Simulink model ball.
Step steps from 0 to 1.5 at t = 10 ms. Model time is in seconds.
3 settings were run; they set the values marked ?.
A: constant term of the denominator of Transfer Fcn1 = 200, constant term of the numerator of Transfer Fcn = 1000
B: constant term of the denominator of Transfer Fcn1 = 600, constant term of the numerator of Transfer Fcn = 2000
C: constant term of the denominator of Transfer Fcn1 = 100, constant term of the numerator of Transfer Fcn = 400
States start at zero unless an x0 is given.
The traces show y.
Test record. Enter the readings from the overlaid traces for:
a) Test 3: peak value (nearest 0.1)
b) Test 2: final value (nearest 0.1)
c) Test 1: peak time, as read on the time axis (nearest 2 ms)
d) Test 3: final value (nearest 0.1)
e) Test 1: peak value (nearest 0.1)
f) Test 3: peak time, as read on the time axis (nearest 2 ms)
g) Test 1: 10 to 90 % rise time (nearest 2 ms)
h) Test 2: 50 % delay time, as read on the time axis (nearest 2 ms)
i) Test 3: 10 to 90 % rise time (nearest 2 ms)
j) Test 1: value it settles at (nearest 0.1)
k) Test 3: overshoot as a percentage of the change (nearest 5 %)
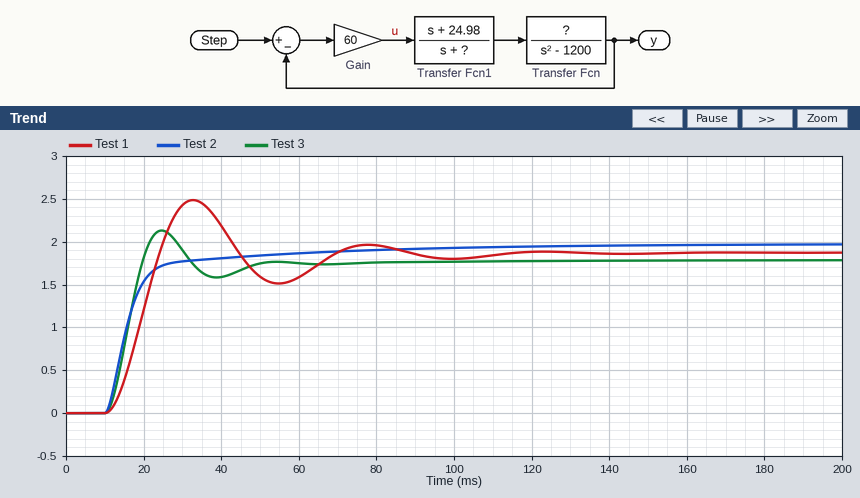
2.1
2.0
32 ms
1.8
2.5
24 ms
10 ms
16 ms
6 ms
1.9
20 %
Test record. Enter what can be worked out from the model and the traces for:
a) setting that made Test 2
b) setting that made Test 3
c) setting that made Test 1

B
A
C
